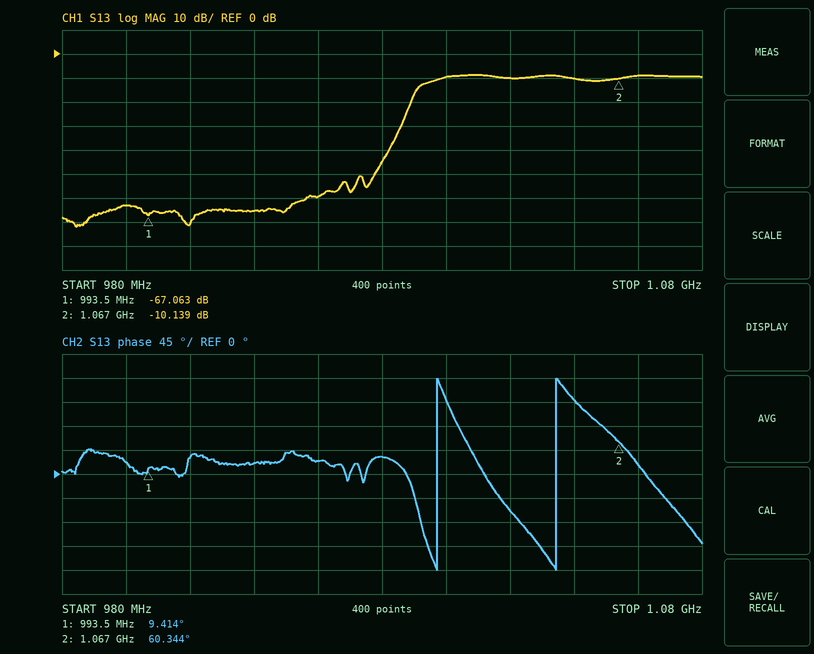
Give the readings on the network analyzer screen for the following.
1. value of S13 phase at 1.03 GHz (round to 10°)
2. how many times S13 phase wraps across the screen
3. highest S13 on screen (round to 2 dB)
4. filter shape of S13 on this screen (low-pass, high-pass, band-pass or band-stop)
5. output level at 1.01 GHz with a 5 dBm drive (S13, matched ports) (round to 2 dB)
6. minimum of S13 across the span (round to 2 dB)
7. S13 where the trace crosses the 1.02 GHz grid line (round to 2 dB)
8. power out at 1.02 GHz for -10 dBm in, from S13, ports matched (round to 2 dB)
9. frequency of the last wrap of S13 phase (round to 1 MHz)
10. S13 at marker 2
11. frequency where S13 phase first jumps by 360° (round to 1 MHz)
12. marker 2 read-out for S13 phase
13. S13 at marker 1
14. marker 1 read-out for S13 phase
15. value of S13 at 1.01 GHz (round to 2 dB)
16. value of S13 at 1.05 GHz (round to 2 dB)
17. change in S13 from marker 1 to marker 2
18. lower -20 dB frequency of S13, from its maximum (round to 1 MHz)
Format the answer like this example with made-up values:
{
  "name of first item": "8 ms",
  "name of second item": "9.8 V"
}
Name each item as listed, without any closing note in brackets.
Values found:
{
  "value of S13 phase at 1.03 GHz": "30°",
  "how many times S13 phase wraps across the screen": "2",
  "highest S13 on screen": "-8 dB",
  "filter shape of S13 on this screen": "high-pass",
  "output level at 1.01 GHz with a 5 dBm drive (S13, matched ports)": "-60 dBm",
  "minimum of S13 across the span": "-72 dB",
  "S13 where the trace crosses the 1.02 GHz grid line": "-60 dB",
  "power out at 1.02 GHz for -10 dBm in, from S13, ports matched": "-70 dBm",
  "frequency of the last wrap of S13 phase": "1.057 GHz",
  "S13 at marker 2": "-10.139 dB",
  "frequency where S13 phase first jumps by 360°": "1.039 GHz",
  "marker 2 read-out for S13 phase": "60.344°",
  "S13 at marker 1": "-67.063 dB",
  "marker 1 read-out for S13 phase": "9.414°",
  "value of S13 at 1.01 GHz": "-66 dB",
  "value of S13 at 1.05 GHz": "-10 dB",
  "change in S13 from marker 1 to marker 2": "56.924 dB",
  "lower -20 dB frequency of S13, from its maximum": "1.033 GHz"
}
